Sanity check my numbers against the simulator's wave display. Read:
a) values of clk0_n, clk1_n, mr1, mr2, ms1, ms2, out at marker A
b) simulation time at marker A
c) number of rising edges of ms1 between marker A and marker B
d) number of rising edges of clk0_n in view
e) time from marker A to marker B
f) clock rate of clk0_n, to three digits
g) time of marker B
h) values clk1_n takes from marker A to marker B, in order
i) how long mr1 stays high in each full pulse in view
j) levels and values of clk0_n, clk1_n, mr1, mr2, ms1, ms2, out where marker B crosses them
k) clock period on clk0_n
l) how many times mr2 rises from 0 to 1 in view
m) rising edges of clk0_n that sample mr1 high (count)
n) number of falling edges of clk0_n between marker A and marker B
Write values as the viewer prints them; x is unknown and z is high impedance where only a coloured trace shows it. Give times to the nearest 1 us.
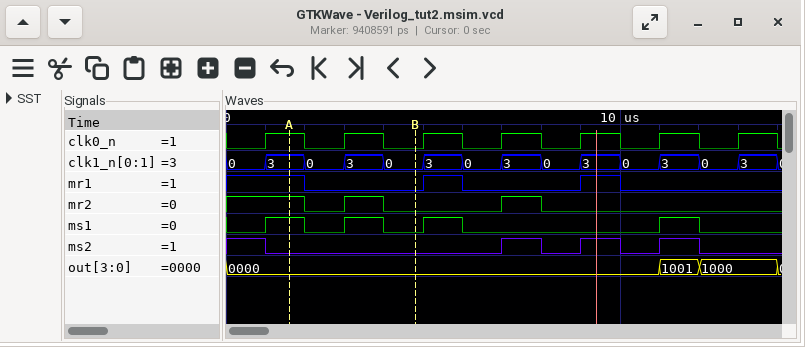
clk0_n=1, clk1_n=3, mr1=1, mr2=1, ms1=1, ms2=0, out=0000
2 us
1
7
3 us
500 kHz
5 us
3, 0, 3, 0
1 us, 1 us
clk0_n=0, clk1_n=0, mr1=0, mr2=0, ms1=0, ms2=0, out=0000
2 us
2
1
2
